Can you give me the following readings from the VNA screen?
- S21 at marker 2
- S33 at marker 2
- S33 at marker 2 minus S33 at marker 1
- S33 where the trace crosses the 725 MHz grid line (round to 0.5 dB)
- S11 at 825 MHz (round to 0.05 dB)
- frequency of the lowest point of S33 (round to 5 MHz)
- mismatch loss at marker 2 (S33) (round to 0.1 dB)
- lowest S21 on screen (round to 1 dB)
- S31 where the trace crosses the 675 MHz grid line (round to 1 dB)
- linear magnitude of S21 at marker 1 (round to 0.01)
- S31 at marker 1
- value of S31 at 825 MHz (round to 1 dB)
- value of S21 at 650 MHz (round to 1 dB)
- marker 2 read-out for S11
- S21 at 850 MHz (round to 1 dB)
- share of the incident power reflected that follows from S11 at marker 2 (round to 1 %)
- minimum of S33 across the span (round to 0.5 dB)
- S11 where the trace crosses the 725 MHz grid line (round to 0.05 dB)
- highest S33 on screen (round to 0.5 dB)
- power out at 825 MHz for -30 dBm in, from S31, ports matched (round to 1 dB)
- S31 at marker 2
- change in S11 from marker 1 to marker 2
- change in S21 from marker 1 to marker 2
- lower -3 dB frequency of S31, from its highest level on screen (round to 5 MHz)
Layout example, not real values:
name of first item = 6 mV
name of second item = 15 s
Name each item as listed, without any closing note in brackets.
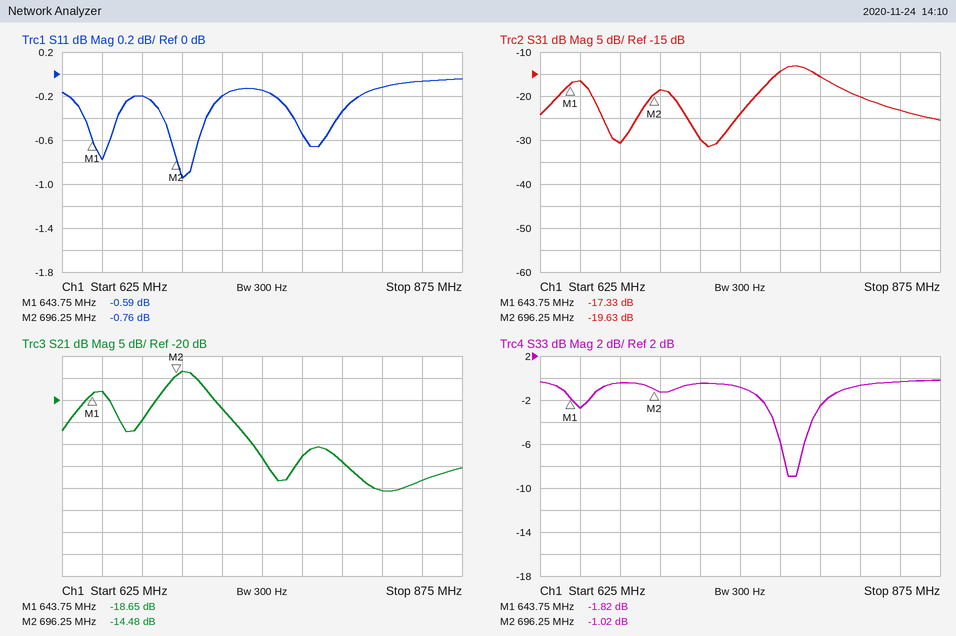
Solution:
S21 at marker 2 = -14.48 dB
S33 at marker 2 = -1.02 dB
S33 at marker 2 minus S33 at marker 1 = 0.80 dB
S33 where the trace crosses the 725 MHz grid line = -0.5 dB
S11 at 825 MHz = -0.10 dB
frequency of the lowest point of S33 = 780 MHz
mismatch loss at marker 2 (S33) = 6.8 dB
lowest S21 on screen = -41 dB
S31 where the trace crosses the 675 MHz grid line = -31 dB
linear magnitude of S21 at marker 1 = 0.12
S31 at marker 1 = -17.33 dB
value of S31 at 825 MHz = -20 dB
value of S21 at 650 MHz = -18 dB
marker 2 read-out for S11 = -0.76 dB
S21 at 850 MHz = -38 dB
share of the incident power reflected that follows from S11 at marker 2 = 84 %
minimum of S33 across the span = -9.0 dB
S11 where the trace crosses the 725 MHz grid line = -0.20 dB
highest S33 on screen = 0.0 dB
power out at 825 MHz for -30 dBm in, from S31, ports matched = -50 dBm
S31 at marker 2 = -19.63 dB
change in S11 from marker 1 to marker 2 = -0.17 dB
change in S21 from marker 1 to marker 2 = 4.17 dB
lower -3 dB frequency of S31, from its highest level on screen = 770 MHz
